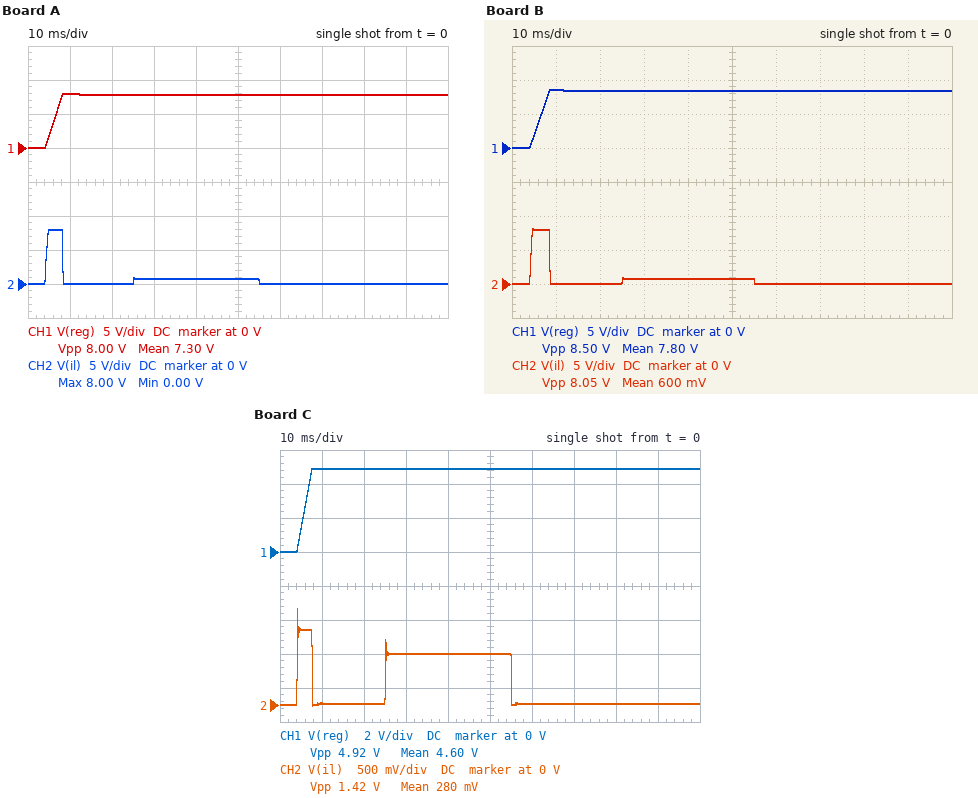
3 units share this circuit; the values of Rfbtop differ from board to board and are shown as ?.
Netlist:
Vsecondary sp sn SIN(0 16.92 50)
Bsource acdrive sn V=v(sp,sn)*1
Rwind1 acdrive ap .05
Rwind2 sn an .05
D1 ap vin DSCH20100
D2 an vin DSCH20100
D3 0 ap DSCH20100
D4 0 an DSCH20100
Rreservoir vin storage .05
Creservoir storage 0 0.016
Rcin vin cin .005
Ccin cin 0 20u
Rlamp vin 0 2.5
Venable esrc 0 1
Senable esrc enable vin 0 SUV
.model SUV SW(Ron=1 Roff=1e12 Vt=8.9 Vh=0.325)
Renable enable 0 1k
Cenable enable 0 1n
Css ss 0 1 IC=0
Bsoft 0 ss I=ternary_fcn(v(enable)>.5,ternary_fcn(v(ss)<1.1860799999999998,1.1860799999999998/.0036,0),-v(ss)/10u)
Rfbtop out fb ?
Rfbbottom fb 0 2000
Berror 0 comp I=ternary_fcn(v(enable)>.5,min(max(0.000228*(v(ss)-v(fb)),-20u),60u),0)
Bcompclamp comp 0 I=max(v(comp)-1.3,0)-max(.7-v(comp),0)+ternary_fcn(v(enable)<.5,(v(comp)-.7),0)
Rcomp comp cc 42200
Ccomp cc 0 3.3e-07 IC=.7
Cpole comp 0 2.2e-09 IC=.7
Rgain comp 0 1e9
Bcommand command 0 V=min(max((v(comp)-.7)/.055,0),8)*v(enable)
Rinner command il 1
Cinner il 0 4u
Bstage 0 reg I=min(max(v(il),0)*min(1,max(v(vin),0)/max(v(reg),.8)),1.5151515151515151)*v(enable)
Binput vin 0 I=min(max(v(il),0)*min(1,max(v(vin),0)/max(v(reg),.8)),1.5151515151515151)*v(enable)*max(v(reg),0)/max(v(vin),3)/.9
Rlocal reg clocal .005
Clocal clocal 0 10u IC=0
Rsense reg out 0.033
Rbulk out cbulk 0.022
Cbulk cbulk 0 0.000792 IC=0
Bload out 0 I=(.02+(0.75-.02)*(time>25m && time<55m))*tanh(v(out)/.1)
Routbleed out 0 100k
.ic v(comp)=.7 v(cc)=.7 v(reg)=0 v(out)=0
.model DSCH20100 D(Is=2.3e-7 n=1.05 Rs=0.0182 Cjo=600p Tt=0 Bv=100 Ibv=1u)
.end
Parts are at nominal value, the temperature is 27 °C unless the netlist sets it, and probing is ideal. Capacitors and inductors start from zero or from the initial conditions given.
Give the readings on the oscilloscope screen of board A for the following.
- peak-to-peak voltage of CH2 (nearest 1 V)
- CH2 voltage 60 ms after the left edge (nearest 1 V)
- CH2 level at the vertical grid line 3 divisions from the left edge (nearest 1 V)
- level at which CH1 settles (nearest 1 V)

8 V
0 V
1 V
8 V
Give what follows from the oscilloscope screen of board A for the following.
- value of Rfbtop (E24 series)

11 kΩ
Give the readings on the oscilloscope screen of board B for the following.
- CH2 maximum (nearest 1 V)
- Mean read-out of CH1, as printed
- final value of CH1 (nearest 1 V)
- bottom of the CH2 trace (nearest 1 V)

8 V
7.80 V
8 V
0 V
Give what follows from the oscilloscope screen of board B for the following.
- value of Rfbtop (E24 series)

12 kΩ
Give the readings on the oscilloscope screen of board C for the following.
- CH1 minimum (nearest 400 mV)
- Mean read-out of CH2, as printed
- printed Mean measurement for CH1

0 V
280 mV
4.60 V
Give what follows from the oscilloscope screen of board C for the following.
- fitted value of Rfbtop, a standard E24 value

6.2 kΩ
